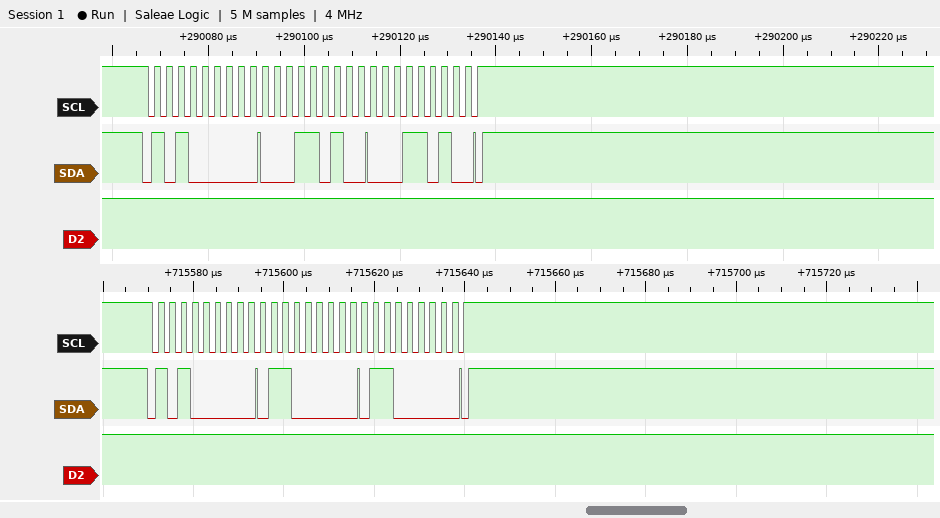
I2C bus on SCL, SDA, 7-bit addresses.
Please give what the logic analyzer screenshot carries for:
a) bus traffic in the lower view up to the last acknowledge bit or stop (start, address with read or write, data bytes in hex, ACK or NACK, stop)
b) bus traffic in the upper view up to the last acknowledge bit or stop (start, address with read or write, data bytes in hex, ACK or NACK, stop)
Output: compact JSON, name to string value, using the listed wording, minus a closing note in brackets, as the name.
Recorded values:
{"bus traffic in the lower view up to the last acknowledge bit or stop": "start, address 50 write ACK, 60 ACK, 60 ACK, stop", "bus traffic in the upper view up to the last acknowledge bit or stop": "start, address 50 write ACK, 1A ACK, 1A ACK, stop"}
